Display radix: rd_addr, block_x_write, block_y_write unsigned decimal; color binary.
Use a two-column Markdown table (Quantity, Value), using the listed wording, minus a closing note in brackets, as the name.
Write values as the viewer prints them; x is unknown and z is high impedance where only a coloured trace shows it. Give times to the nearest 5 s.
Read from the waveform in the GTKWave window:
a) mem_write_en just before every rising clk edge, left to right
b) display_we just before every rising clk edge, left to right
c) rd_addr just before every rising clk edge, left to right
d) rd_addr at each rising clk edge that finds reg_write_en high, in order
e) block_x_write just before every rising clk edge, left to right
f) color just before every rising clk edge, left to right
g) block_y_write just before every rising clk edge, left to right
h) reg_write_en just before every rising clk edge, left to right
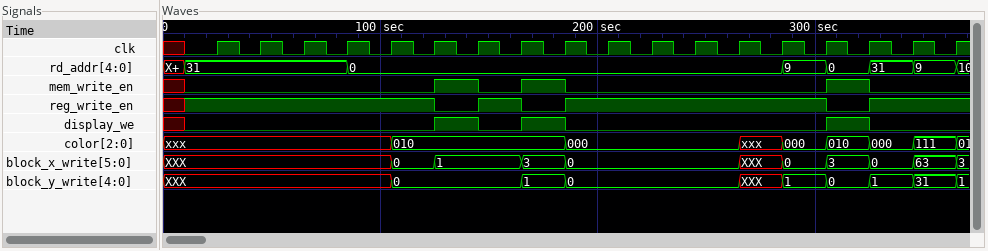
| Quantity | Value |
|---|---|
| mem_write_en just before every rising clk edge, left to right | 0 0 0 0 0 0 1 0 1 0 0 0 0 0 0 1 0 0 |
| display_we just before every rising clk edge, left to right | 0 0 0 0 0 0 1 0 1 0 0 0 0 0 0 1 0 0 |
| rd_addr just before every rising clk edge, left to right | 31, 31, 31, 31, 0, 0, 0, 0, 0, 0, 0, 0, 0, 0, 9, 0, 31, 9 |
| rd_addr at each rising clk edge that finds reg_write_en high, in order | 31, 31, 31, 31, 0, 0, 0, 0, 0, 0, 0, 0, 9, 31, 9 |
| block_x_write just before every rising clk edge, left to right | XXX, XXX, XXX, XXX, XXX, 0, 1, 1, 3, 0, 0, 0, 0, XXX, 0, 3, 0, 63 |
| color just before every rising clk edge, left to right | xxx, xxx, xxx, xxx, xxx, 010, 010, 010, 010, 000, 000, 000, 000, xxx, 000, 010, 000, 111 |
| block_y_write just before every rising clk edge, left to right | XXX, XXX, XXX, XXX, XXX, 0, 0, 0, 1, 0, 0, 0, 0, XXX, 1, 0, 1, 31 |
| reg_write_en just before every rising clk edge, left to right | 1 1 1 1 1 1 0 1 0 1 1 1 1 1 1 0 1 1 |
